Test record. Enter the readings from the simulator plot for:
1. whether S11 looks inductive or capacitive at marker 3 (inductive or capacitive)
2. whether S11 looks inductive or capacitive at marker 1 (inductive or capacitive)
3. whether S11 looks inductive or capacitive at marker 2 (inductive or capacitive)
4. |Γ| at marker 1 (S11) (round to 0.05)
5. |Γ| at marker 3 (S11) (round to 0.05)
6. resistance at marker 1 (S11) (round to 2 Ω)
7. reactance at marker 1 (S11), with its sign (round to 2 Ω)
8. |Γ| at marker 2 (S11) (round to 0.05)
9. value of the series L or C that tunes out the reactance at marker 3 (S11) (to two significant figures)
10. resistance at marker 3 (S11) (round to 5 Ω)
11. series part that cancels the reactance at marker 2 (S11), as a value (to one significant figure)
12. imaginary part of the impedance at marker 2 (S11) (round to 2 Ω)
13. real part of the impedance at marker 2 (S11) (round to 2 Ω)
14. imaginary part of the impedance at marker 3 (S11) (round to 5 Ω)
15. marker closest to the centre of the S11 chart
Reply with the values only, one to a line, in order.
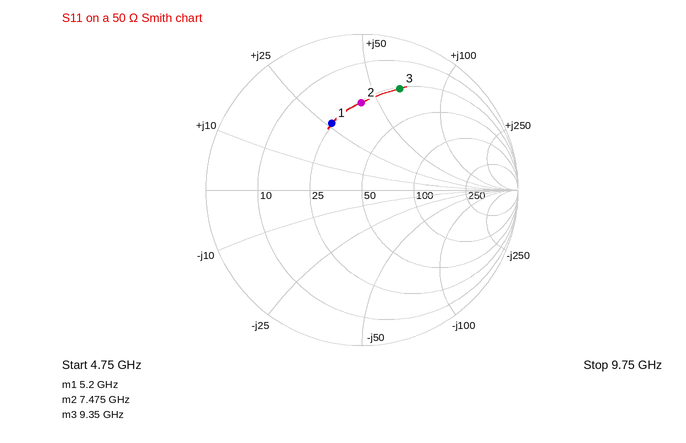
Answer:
inductive
inductive
inductive
0.45
0.70
24 Ω
+26 Ω
0.55
260 fF
25 Ω
500 fF
+42 Ω
26 Ω
+65 Ω
marker 1
